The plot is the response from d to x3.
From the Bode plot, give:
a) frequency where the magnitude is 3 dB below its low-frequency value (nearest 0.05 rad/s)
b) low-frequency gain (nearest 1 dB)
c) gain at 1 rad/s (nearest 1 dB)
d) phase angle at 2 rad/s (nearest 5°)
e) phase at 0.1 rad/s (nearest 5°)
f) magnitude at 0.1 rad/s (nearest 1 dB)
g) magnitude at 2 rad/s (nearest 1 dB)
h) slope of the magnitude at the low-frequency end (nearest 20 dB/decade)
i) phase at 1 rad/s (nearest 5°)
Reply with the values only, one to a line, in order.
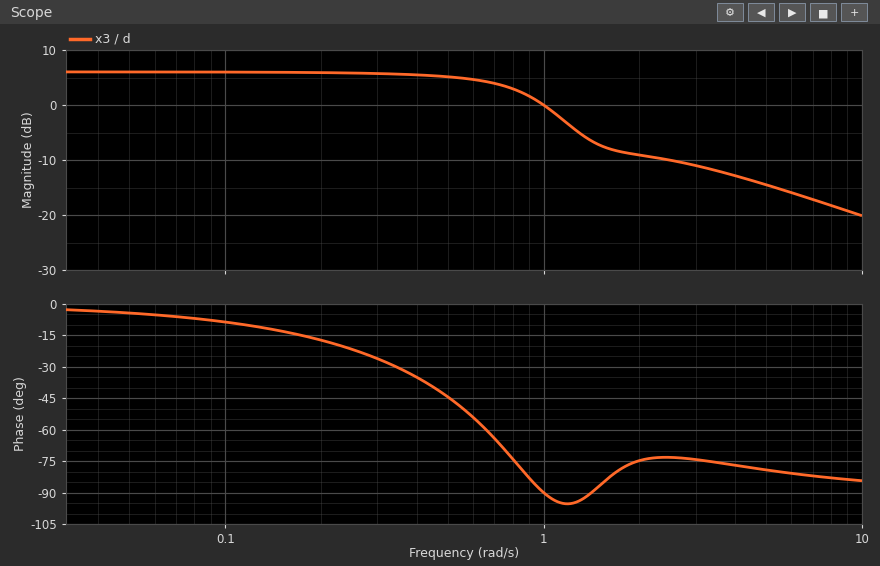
0.80 rad/s
6 dB
0 dB
-75°
-10°
6 dB
-9 dB
0 dB/decade
-90°
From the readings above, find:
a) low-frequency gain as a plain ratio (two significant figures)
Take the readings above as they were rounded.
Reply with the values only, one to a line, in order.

2.0
